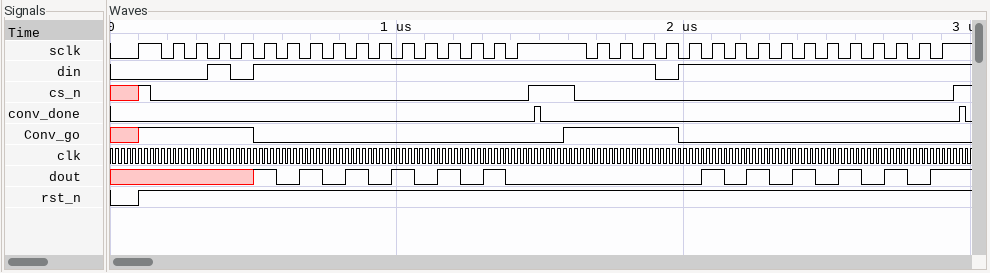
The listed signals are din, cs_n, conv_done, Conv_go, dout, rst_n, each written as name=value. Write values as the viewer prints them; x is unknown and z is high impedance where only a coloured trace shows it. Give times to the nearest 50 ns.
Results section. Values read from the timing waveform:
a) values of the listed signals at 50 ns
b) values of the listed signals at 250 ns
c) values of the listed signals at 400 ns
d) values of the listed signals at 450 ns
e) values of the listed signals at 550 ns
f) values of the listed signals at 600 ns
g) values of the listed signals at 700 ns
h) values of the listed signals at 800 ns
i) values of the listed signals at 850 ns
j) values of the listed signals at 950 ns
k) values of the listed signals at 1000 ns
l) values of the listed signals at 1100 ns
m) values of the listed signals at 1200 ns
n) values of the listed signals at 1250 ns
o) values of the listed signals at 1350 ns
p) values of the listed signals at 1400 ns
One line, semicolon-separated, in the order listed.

din=0, cs_n=x, conv_done=0, Conv_go=x, dout=x, rst_n=0; din=0, cs_n=0, conv_done=0, Conv_go=1, dout=x, rst_n=1; din=1, cs_n=0, conv_done=0, Conv_go=1, dout=x, rst_n=1; din=0, cs_n=0, conv_done=0, Conv_go=1, dout=x, rst_n=1; din=1, cs_n=0, conv_done=0, Conv_go=0, dout=1, rst_n=1; din=1, cs_n=0, conv_done=0, Conv_go=0, dout=0, rst_n=1; din=1, cs_n=0, conv_done=0, Conv_go=0, dout=1, rst_n=1; din=1, cs_n=0, conv_done=0, Conv_go=0, dout=0, rst_n=1; din=1, cs_n=0, conv_done=0, Conv_go=0, dout=1, rst_n=1; din=1, cs_n=0, conv_done=0, Conv_go=0, dout=0, rst_n=1; din=1, cs_n=0, conv_done=0, Conv_go=0, dout=1, rst_n=1; din=1, cs_n=0, conv_done=0, Conv_go=0, dout=0, rst_n=1; din=1, cs_n=0, conv_done=0, Conv_go=0, dout=1, rst_n=1; din=1, cs_n=0, conv_done=0, Conv_go=0, dout=0, rst_n=1; din=1, cs_n=0, conv_done=0, Conv_go=0, dout=1, rst_n=1; din=1, cs_n=0, conv_done=0, Conv_go=0, dout=0, rst_n=1
